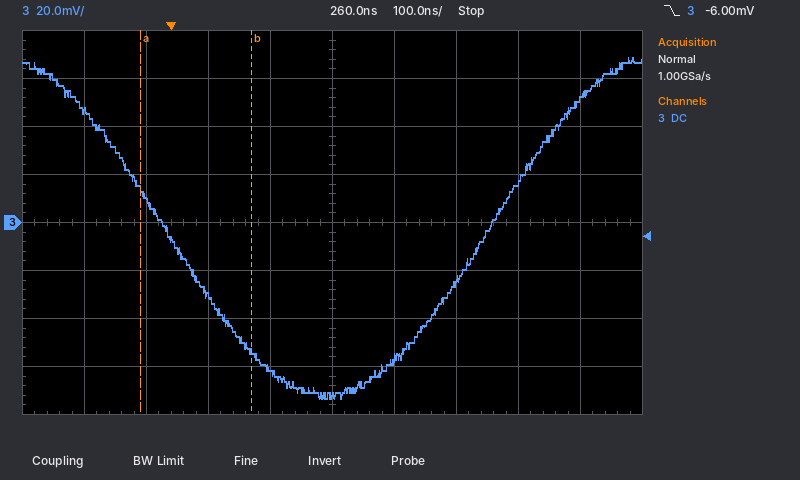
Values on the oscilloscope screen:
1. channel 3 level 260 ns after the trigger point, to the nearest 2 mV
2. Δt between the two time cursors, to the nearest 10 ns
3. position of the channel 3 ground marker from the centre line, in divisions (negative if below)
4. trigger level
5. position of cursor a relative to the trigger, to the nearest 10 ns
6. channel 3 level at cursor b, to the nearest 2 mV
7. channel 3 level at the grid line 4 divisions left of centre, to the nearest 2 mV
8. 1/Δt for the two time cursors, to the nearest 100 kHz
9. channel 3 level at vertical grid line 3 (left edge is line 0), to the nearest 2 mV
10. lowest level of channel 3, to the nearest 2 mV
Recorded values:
-72 mV
180 ns
0.0 div
-6.00 mV
-50 ns
-54 mV
46 mV
5.6 MHz
-30 mV
-74 mV
